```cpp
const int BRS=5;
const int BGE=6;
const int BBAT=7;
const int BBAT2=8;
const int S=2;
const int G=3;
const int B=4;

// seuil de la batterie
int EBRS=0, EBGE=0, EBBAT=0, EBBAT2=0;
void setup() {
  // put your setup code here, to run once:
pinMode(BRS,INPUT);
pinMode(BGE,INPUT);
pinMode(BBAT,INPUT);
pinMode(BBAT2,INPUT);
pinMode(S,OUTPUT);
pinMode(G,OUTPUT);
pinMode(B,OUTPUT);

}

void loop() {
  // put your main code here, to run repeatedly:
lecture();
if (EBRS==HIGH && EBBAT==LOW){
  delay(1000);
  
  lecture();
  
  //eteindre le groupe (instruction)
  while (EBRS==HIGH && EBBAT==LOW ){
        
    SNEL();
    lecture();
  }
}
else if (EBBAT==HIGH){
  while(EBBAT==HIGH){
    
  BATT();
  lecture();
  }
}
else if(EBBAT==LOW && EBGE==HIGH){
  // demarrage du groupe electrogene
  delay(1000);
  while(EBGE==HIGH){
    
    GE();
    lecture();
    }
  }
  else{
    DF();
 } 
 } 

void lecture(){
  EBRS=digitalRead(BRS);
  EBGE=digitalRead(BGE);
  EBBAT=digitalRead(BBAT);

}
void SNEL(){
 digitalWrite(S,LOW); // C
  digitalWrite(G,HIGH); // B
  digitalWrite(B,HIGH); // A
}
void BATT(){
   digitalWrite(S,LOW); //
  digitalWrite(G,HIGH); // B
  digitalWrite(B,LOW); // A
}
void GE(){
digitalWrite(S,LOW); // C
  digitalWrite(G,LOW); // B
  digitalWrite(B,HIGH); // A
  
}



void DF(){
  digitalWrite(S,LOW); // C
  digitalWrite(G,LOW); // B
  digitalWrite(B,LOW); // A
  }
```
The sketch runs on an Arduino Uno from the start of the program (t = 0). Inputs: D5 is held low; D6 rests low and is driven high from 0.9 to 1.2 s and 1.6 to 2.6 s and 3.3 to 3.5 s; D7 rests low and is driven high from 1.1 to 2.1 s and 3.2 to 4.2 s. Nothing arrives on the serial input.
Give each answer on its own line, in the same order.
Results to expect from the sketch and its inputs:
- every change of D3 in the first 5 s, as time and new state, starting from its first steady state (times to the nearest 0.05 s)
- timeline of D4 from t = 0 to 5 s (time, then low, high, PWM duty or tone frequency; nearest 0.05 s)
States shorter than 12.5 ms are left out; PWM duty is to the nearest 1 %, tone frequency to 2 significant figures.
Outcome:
0 s low; 3.2 s high; 4.2 s low
0 s low; 1.9 s high; 2.6 s low
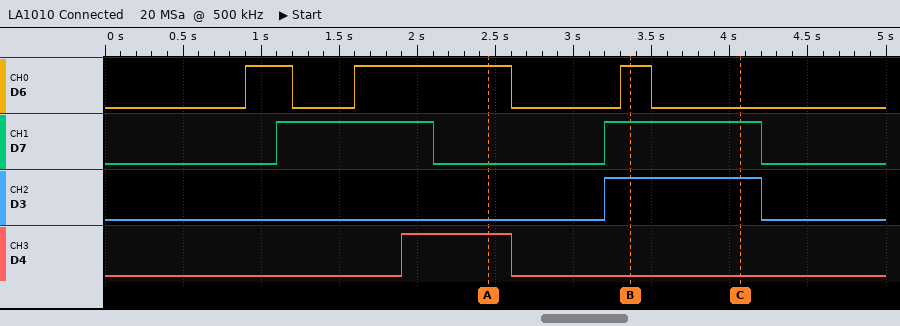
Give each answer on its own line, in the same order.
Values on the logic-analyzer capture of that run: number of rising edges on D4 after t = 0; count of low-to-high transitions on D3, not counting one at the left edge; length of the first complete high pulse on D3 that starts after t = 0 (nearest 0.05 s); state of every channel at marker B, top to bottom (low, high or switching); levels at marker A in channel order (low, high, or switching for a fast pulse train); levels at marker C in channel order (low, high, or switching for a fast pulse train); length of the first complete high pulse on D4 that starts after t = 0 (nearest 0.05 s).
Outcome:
1
1
1.00 s
D6 high, D7 high, D3 high, D4 low
D6 high, D7 low, D3 low, D4 high
D6 low, D7 high, D3 high, D4 low
0.70 s
